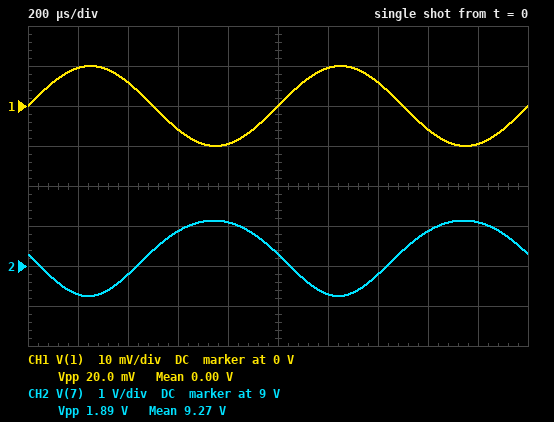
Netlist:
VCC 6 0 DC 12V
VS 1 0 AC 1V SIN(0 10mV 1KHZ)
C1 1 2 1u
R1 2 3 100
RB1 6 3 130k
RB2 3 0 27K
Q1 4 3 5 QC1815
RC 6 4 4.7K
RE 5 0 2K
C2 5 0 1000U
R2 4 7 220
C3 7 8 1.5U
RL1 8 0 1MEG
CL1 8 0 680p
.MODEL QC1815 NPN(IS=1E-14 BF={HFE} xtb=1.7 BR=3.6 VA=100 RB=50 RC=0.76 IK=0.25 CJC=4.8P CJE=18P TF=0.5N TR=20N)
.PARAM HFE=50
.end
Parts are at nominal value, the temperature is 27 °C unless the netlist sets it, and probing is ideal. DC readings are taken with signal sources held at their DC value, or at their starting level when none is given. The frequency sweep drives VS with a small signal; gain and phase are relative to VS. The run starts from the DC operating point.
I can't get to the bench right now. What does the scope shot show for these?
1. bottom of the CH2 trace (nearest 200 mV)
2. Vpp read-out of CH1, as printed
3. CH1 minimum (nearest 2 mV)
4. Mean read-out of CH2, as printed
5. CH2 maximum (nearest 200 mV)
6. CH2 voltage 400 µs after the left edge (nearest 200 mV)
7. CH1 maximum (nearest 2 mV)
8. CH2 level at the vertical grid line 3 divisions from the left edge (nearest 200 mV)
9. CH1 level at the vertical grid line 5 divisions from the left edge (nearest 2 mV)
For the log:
8.2 V
20.0 mV
-10 mV
9.27 V
10.2 V
8.8 V
10 mV
9.8 V
0 V
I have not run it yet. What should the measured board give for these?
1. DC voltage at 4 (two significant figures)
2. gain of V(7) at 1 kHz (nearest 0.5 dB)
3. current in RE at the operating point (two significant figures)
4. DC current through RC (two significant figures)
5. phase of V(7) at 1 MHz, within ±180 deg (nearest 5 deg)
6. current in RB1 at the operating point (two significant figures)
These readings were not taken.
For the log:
9.3 V
39.5 dB
590 µA
580 µA
90 deg
78 µA
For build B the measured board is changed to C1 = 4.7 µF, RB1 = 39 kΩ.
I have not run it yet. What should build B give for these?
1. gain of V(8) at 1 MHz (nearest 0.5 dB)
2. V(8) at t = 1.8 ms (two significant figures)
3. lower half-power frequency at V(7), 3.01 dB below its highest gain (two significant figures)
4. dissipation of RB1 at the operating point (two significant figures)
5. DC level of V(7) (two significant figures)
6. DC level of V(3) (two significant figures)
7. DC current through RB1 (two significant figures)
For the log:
17.5 dB
2.3 V
150 Hz
1.5 mW
3.7 V
4.3 V
200 µA
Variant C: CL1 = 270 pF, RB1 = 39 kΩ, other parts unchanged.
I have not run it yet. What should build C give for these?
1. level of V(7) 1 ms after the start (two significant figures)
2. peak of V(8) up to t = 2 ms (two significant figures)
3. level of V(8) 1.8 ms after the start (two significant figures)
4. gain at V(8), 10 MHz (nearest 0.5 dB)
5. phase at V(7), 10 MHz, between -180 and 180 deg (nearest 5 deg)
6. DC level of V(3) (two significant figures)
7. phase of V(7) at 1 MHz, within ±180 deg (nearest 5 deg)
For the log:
3.7 V
2.5 V
2.2 V
-1.0 dB
35 deg
4.3 V
115 deg
